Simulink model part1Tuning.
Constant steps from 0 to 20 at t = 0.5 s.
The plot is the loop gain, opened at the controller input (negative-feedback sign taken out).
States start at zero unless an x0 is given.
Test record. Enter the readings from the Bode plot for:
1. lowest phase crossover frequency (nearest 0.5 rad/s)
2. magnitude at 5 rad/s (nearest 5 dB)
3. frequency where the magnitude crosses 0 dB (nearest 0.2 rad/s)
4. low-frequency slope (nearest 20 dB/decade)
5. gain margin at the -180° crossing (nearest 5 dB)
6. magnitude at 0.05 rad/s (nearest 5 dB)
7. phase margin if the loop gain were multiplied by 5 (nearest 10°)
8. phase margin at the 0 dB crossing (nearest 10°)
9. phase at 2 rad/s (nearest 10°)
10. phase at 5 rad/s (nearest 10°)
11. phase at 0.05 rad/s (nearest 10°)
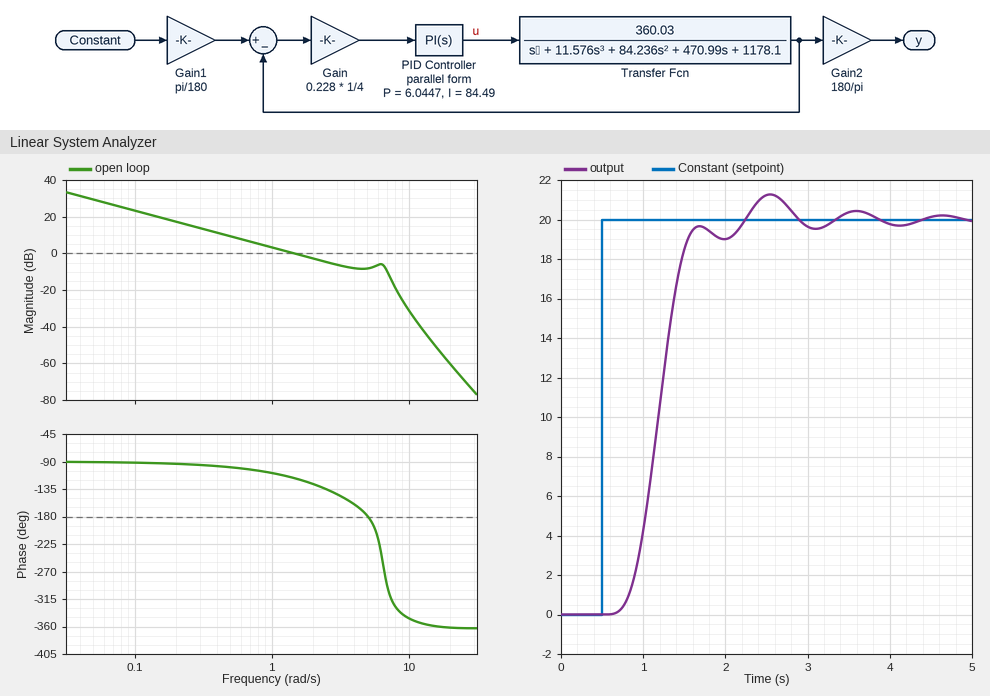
5.0 rad/s
-10 dB
1.4 rad/s
-20 dB/decade
10 dB
30 dB
-130°
60°
-130°
-180°
-90°
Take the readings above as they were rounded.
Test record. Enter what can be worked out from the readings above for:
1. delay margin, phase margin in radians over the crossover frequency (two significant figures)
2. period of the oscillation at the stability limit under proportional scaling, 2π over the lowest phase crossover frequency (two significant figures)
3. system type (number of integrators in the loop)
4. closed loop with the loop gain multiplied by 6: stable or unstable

0.75 s
1.3 s
1
unstable
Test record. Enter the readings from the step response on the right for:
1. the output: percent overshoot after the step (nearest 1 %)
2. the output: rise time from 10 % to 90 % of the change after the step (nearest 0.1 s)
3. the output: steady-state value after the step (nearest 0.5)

6 %
0.6 s
20.0
